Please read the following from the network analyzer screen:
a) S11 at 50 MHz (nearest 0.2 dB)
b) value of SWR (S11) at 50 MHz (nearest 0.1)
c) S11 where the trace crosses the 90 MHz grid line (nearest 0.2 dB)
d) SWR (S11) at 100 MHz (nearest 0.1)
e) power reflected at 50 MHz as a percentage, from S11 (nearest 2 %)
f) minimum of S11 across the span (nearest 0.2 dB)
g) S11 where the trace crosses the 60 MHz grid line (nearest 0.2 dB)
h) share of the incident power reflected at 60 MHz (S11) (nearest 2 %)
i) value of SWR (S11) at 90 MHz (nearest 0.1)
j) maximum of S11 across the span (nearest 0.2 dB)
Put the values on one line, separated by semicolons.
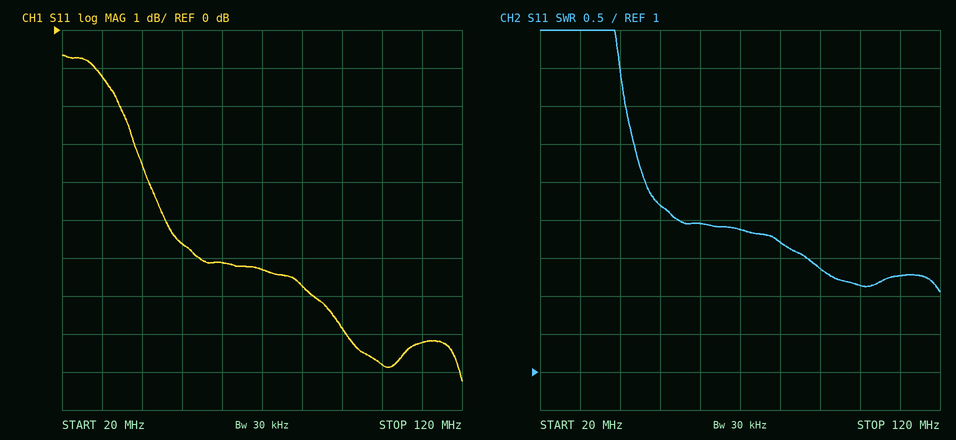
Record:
-5.6 dB; 3.2; -7.8 dB; 2.1; 28 %; -9.2 dB; -6.2 dB; 24 %; 2.4; -0.6 dB
